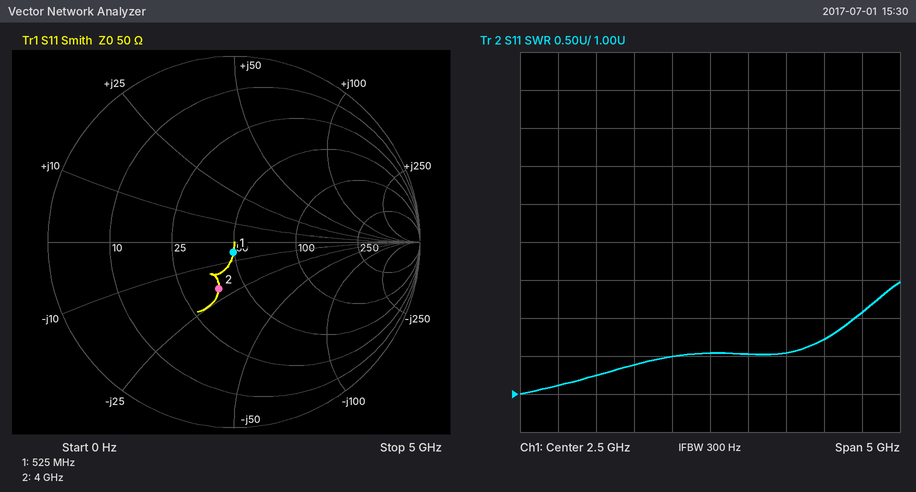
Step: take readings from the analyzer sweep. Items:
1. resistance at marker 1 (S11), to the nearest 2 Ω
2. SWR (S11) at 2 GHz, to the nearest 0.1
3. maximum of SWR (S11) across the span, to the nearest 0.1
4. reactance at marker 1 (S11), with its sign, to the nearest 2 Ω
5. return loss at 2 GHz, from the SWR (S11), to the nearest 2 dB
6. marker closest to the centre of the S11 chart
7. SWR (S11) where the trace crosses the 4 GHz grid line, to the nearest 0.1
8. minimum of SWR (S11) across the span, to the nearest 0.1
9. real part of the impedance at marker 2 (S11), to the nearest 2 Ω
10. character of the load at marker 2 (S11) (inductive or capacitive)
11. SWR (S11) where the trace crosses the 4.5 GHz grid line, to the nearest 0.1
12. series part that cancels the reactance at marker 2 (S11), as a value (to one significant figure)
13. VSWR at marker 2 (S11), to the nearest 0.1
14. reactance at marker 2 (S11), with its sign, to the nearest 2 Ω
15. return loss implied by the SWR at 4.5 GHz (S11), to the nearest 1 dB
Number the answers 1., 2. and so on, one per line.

1. 50 Ω
2. 1.5
3. 2.5
4. -6 Ω
5. 14 dB
6. marker 1
7. 1.7
8. 1.0
9. 38 Ω
10. capacitive
11. 2.1
12. 800 pH
13. 1.7
14. -20 Ω
15. 9 dB
